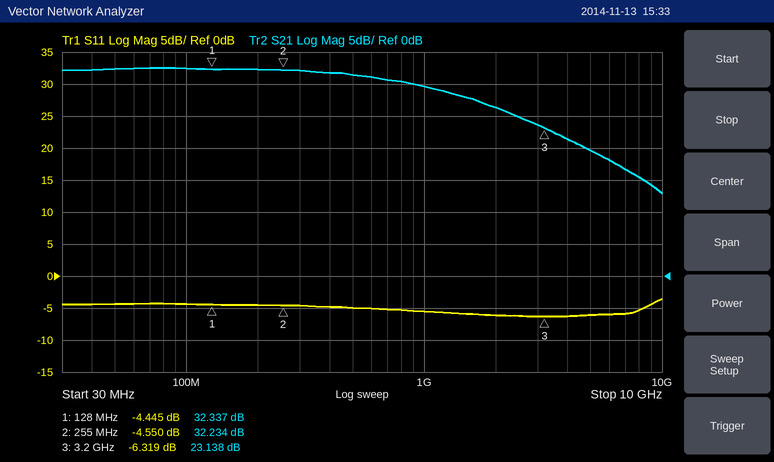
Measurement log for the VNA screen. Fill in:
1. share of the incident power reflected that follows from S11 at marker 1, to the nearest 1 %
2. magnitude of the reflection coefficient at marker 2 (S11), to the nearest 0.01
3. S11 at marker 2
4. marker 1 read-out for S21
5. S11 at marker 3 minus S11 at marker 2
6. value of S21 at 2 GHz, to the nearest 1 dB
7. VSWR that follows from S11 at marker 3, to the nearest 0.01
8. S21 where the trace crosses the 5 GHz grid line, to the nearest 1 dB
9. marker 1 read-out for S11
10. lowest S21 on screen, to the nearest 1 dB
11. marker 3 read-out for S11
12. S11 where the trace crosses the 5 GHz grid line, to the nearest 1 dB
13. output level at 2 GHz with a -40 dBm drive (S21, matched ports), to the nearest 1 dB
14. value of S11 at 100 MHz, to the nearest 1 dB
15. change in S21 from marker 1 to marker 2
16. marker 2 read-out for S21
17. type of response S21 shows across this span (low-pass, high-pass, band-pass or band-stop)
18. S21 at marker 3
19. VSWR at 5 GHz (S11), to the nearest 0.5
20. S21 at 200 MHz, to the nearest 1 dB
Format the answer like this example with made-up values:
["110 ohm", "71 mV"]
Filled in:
["36 %", "0.59", "-4.550 dB", "32.337 dB", "-1.769 dB", "26 dB", "2.87", "20 dB", "-4.445 dB", "13 dB", "-6.319 dB", "-6 dB", "-14 dBm", "-4 dB", "-0.103 dB", "32.234 dB", "low-pass", "23.138 dB", "3.0", "32 dB"]
